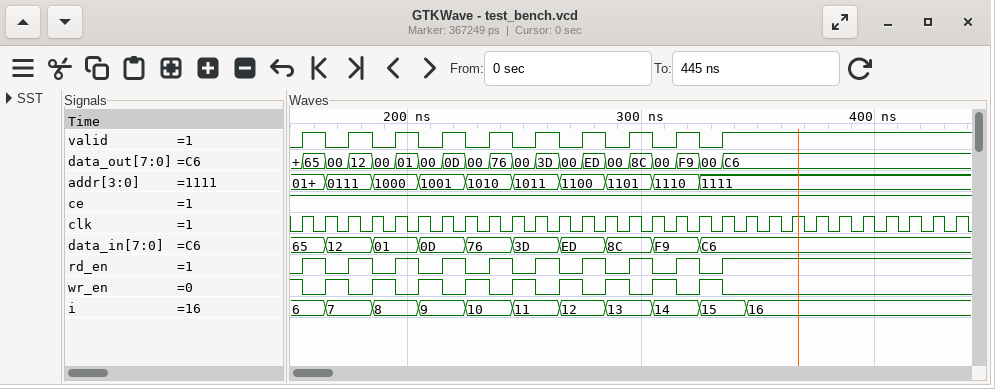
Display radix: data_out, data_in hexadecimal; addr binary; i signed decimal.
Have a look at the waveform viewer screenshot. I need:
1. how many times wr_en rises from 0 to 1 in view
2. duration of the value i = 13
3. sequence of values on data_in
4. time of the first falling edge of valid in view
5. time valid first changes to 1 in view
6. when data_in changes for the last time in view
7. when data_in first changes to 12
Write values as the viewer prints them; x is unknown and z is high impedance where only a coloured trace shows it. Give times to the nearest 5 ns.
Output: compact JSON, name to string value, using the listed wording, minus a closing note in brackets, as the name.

{"how many times wr_en rises from 0 to 1 in view": "9", "duration of the value i = 13": "20 ns", "sequence of values on data_in": "65, 12, 01, 0D, 76, 3D, ED, 8C, F9, C6", "time of the first falling edge of valid in view": "165 ns", "time valid first changes to 1 in view": "155 ns", "when data_in changes for the last time in view": "325 ns", "when data_in first changes to 12": "165 ns"}
